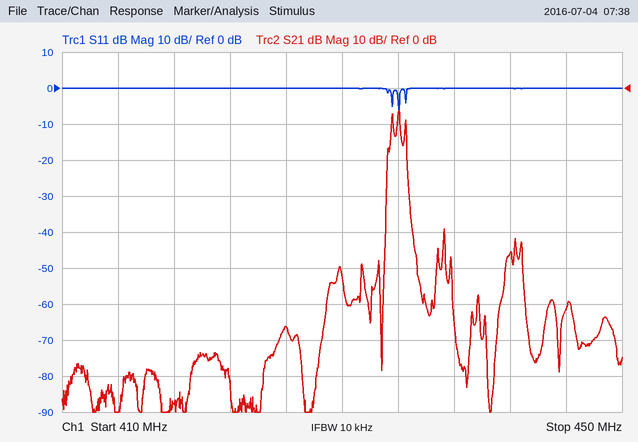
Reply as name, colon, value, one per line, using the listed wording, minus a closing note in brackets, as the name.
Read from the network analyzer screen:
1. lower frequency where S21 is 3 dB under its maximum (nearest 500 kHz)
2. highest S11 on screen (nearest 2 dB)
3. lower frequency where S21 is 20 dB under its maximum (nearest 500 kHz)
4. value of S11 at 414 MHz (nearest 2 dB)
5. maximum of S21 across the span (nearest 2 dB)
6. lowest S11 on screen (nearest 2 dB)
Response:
lower frequency where S21 is 3 dB under its maximum: 434.0 MHz
highest S11 on screen: 0 dB
lower frequency where S21 is 20 dB under its maximum: 433.0 MHz
value of S11 at 414 MHz: 0 dB
maximum of S21 across the span: -6 dB
lowest S11 on screen: -6 dB
